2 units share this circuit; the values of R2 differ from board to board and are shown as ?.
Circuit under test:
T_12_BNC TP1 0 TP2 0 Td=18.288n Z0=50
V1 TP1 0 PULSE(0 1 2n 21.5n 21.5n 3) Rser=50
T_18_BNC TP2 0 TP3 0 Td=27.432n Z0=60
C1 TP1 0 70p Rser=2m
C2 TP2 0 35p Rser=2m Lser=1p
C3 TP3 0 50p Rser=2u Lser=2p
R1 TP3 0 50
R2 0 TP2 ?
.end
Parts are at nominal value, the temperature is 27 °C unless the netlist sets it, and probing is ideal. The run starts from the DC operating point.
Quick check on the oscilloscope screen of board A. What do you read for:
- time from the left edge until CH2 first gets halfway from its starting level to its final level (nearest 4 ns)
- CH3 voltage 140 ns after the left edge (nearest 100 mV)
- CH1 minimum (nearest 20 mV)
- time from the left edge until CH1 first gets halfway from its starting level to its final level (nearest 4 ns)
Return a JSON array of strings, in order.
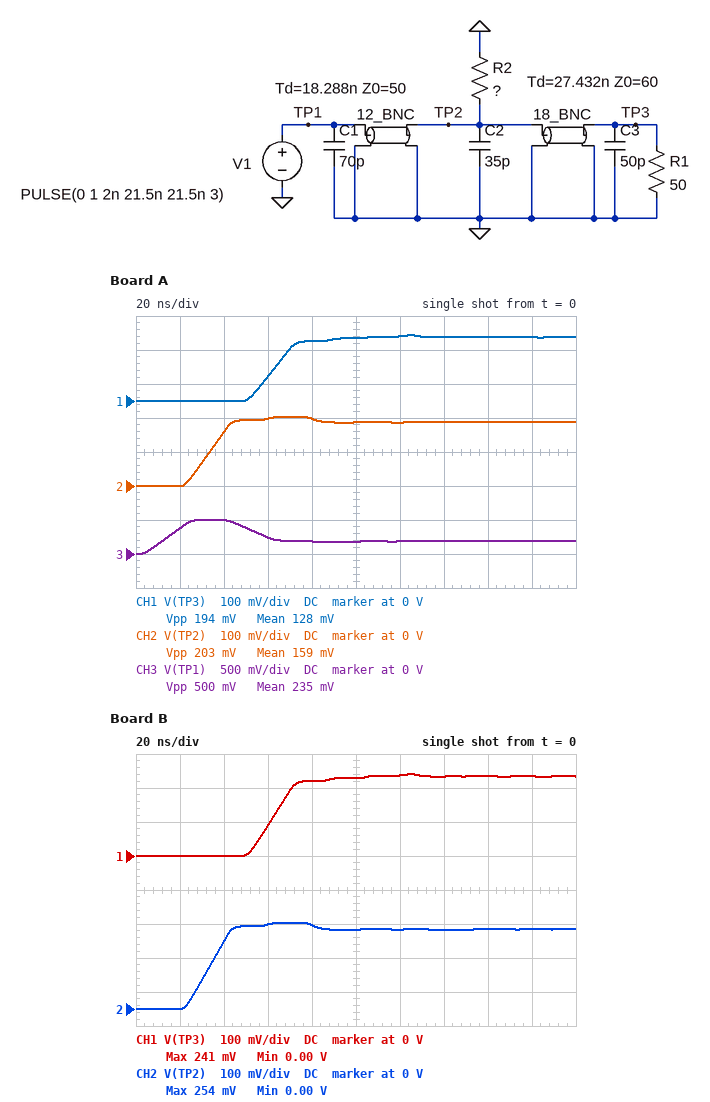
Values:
["32 ns", "200 mV", "0 V", "64 ns"]
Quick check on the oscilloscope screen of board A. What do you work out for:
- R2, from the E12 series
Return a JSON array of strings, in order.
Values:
["15 Ω"]
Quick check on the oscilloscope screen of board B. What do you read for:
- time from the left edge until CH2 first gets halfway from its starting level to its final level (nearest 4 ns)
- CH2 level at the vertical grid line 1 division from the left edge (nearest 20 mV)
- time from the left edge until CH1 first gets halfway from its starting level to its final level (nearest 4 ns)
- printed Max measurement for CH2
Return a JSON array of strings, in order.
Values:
["32 ns", "0 V", "64 ns", "254 mV"]
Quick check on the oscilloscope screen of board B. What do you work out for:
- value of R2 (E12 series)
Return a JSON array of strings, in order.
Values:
["22 Ω"]
